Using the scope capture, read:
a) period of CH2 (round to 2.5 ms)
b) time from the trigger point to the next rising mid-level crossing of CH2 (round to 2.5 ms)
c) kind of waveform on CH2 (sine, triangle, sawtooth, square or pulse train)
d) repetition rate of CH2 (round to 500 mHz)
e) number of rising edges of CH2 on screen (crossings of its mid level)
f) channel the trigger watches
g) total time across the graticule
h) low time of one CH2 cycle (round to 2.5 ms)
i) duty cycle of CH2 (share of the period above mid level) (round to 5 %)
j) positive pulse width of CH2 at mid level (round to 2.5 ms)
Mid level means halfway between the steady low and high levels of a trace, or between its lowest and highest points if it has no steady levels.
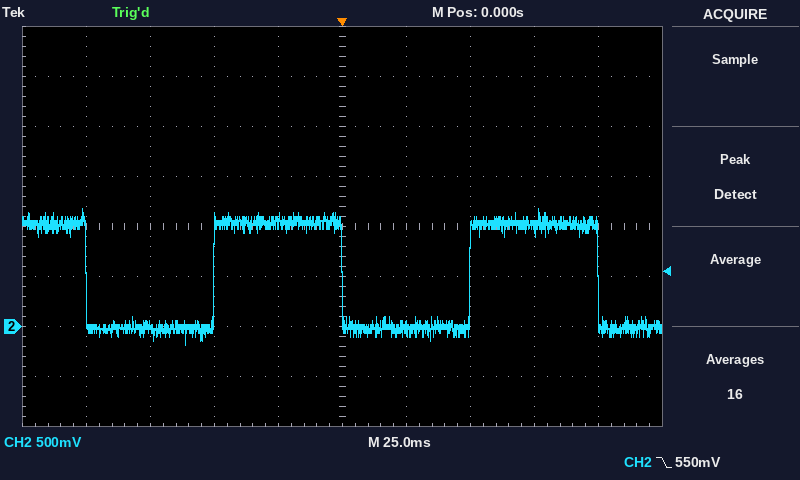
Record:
100.0 ms
50.0 ms
square
10.0 Hz
2
CH2
250 ms
50.0 ms
50 %
50.0 ms
